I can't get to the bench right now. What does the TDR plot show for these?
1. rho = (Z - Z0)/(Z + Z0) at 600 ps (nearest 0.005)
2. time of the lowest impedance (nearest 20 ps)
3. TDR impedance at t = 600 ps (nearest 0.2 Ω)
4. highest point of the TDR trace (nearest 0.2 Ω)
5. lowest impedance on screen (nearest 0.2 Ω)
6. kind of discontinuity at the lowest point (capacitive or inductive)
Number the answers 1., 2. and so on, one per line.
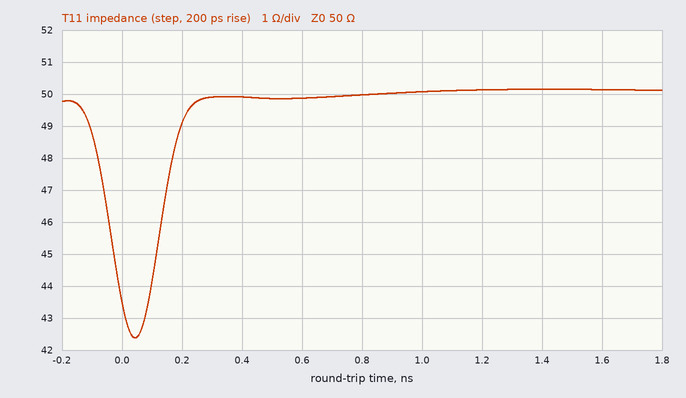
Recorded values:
1. 0.000
2. 40 ps
3. 49.8 Ω
4. 50.2 Ω
5. 42.4 Ω
6. capacitive
